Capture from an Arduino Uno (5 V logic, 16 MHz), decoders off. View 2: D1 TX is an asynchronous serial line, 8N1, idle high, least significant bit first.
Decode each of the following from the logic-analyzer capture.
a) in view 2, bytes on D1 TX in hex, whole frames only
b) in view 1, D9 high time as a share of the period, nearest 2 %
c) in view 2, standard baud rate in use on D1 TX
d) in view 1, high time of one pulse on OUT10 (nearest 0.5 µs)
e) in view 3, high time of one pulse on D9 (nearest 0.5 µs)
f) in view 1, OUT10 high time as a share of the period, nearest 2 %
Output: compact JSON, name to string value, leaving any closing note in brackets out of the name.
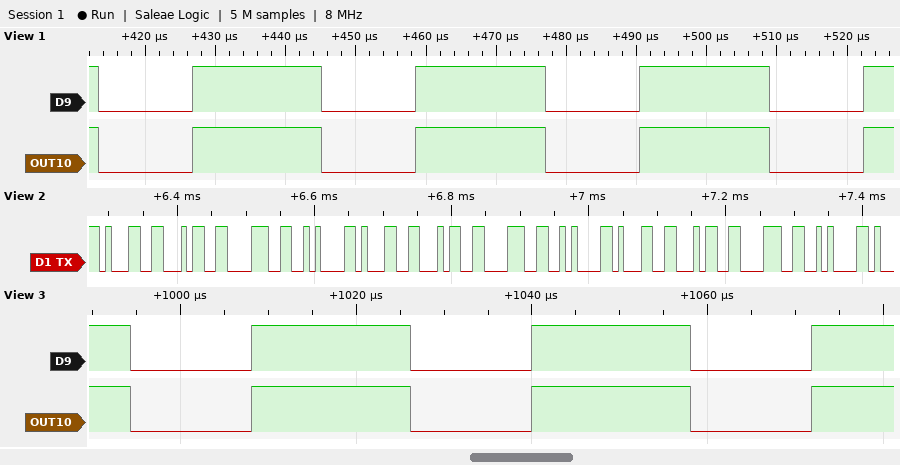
{"in view 2, bytes on D1 TX in hex, whole frames only": "31 34 38 0A 31 34 38 0A 31 34 38 0A", "in view 1, D9 high time as a share of the period, nearest 2 %": "58 %", "in view 2, standard baud rate in use on D1 TX": "115200 baud", "in view 1, high time of one pulse on OUT10": "18.5 µs", "in view 3, high time of one pulse on D9": "18.0 µs", "in view 1, OUT10 high time as a share of the period, nearest 2 %": "58 %"}
